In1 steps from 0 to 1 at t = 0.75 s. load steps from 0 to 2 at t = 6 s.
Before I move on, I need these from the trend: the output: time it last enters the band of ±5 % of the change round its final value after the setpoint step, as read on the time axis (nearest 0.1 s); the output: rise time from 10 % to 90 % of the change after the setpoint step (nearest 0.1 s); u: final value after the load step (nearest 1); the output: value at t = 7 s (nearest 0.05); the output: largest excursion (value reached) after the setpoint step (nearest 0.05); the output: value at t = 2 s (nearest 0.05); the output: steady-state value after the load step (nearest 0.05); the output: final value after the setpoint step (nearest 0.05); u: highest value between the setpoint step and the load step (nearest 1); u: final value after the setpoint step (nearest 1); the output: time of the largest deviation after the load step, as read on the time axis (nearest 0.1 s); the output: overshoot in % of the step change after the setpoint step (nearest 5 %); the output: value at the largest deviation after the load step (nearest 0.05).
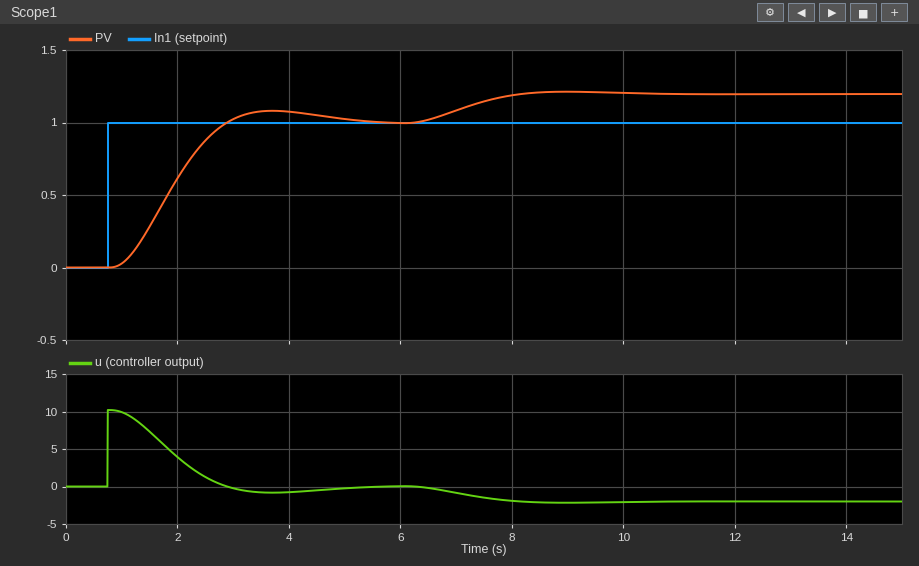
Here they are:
4.5 s
1.4 s
-2
1.10
1.10
0.60
1.20
1.00
10
0
9.0 s
10 %
1.20
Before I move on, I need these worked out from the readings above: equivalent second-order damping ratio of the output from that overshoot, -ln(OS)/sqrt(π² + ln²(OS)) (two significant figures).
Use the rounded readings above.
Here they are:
0.59
